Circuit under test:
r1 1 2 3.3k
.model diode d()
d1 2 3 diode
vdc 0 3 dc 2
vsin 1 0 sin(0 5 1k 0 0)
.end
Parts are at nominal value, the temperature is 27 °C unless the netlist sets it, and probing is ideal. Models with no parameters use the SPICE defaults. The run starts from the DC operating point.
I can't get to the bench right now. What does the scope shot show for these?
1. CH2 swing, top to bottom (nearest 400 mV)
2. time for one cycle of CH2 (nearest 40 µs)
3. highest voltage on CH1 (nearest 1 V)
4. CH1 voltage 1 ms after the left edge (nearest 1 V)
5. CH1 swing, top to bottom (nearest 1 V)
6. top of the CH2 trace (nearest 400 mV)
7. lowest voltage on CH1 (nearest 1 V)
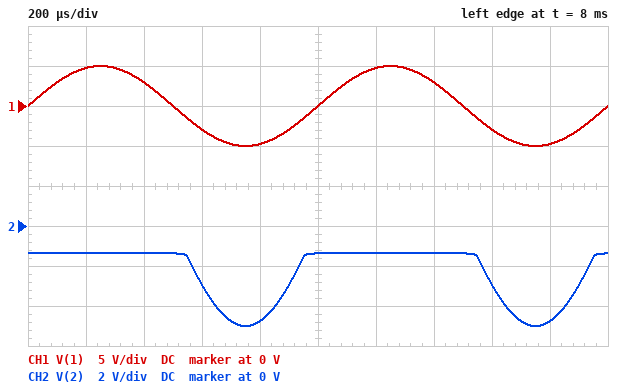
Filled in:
3.6 V
1.00 ms
5 V
0 V
10 V
-1.2 V
-5 V
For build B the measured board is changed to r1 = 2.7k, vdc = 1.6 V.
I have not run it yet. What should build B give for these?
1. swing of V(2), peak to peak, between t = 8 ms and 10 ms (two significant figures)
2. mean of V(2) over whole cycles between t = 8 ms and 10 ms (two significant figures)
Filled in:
4.1 V
-2.1 V
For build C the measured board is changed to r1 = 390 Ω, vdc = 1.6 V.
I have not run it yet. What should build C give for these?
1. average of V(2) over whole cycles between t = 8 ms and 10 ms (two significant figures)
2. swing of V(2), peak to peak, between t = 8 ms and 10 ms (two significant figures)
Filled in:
-2.1 V
4.1 V
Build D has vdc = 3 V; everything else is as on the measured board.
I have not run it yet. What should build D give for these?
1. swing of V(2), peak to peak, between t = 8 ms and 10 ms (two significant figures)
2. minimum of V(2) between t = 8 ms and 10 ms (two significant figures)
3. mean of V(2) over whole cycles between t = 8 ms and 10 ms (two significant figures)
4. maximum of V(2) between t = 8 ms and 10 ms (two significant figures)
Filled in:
2.7 V
-5.0 V
-2.9 V
-2.3 V
